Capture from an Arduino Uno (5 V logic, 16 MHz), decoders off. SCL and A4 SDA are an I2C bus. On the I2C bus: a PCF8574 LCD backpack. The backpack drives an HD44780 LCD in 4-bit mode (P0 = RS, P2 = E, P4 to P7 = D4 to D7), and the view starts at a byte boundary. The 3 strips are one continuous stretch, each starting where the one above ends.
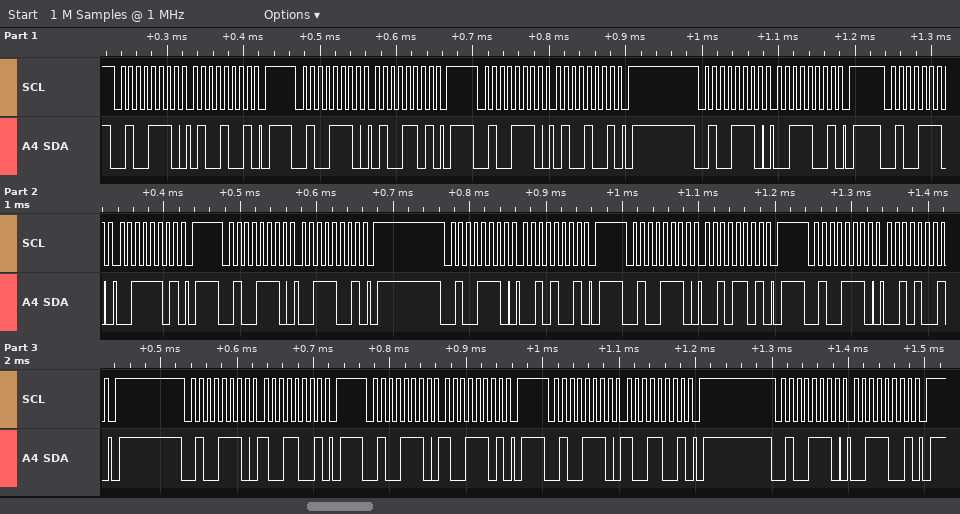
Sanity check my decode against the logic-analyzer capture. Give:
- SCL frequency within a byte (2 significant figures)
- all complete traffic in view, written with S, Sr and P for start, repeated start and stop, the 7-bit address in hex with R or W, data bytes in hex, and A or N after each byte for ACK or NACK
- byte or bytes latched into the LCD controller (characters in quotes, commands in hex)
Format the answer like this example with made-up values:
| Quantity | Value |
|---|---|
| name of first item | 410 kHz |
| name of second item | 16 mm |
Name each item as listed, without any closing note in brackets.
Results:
| Quantity | Value |
|---|---|
| SCL frequency within a byte | 100 kHz |
| all complete traffic in view, written with S, Sr and P for start, repeated start and stop, the 7-bit address in hex with R or W, data bytes in hex, and A or N after each byte for ACK or NACK | S 27W A 49 A P S 27W A 4D A P S 27W A 49 A P S 27W A 39 A P S 27W A 3D A P S 27W A 39 A P S 27W A 29 A P S 27W A 2D A P S 27W A 29 A P S 27W A 99 A P S 27W A 9D A P S 27W A 99 A P S 27W A 39 A P |
| byte or bytes latched into the LCD controller | 'C' ')' |
